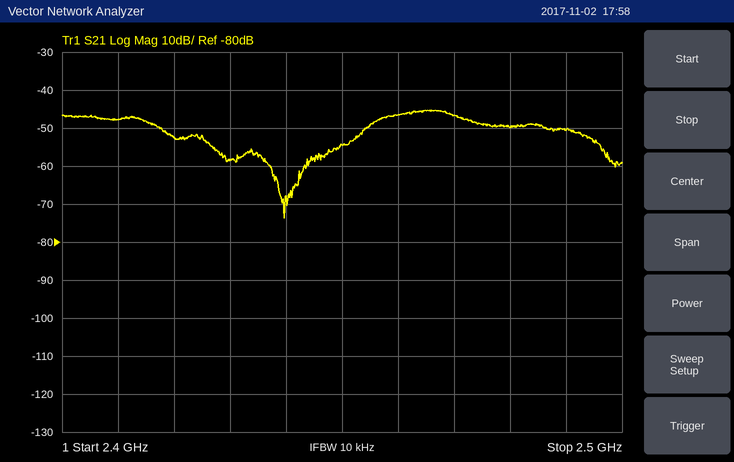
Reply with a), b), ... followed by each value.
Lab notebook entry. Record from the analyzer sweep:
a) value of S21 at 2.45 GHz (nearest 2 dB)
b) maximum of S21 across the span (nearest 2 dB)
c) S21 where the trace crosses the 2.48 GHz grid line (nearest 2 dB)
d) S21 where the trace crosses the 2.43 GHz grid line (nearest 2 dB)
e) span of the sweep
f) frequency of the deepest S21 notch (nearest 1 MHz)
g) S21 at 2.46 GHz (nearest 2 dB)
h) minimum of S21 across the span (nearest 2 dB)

a) -54 dB
b) -46 dB
c) -50 dB
d) -58 dB
e) 100 MHz
f) 2.440 GHz
g) -46 dB
h) -74 dB
